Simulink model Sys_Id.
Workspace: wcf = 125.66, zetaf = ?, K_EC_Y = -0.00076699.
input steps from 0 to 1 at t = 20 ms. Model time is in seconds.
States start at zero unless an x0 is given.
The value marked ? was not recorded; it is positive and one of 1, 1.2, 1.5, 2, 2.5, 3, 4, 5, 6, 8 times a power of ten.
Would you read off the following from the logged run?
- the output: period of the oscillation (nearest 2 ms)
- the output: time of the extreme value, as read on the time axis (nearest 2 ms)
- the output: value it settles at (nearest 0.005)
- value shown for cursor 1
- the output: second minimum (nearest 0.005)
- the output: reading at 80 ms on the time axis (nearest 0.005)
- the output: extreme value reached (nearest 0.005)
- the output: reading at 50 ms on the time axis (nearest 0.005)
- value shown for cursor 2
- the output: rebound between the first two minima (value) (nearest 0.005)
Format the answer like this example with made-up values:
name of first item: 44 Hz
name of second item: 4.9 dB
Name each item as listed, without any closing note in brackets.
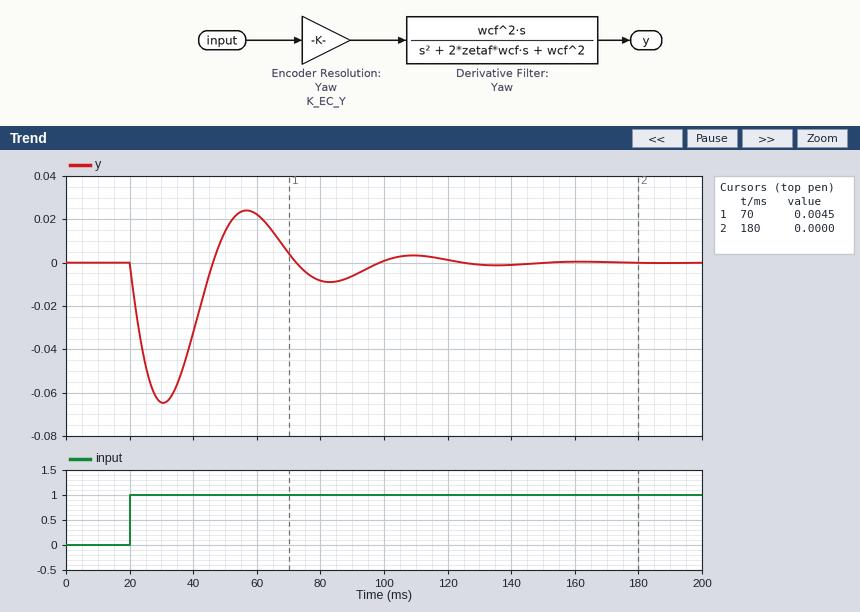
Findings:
the output: period of the oscillation: 52 ms
the output: time of the extreme value, as read on the time axis: 30 ms
the output: value it settles at: 0.000
value shown for cursor 1: 0.0045
the output: second minimum: -0.010
the output: reading at 80 ms on the time axis: -0.010
the output: extreme value reached: -0.065
the output: reading at 50 ms on the time axis: 0.015
value shown for cursor 2: 0.0000
the output: rebound between the first two minima (value): 0.025
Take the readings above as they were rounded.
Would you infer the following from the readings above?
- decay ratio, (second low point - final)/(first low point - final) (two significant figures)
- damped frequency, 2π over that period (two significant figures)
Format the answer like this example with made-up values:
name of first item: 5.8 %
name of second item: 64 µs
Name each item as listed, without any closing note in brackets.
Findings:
decay ratio, (second low point - final)/(first low point - final): 0.15
damped frequency, 2π over that period: 0.12 rad/ms
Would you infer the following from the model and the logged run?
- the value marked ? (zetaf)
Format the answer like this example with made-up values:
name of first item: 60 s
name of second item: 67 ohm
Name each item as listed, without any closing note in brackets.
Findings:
the value marked ?: 0.3
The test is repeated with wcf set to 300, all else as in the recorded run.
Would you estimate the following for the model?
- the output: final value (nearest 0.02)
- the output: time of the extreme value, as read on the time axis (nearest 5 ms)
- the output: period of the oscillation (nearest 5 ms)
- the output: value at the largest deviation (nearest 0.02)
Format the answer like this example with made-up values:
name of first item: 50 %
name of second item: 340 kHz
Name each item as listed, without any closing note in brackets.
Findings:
the output: final value: 0.00
the output: time of the extreme value, as read on the time axis: 25 ms
the output: period of the oscillation: 20 ms
the output: value at the largest deviation: -0.16
